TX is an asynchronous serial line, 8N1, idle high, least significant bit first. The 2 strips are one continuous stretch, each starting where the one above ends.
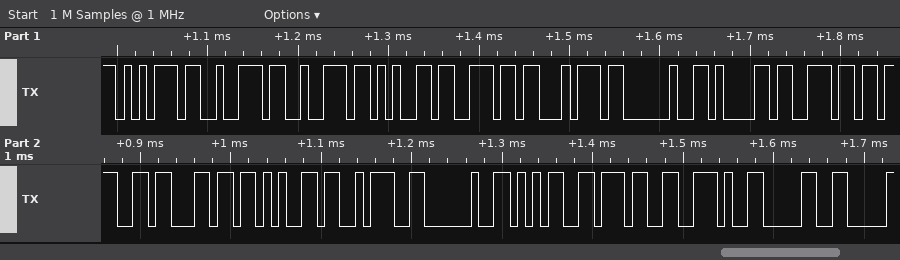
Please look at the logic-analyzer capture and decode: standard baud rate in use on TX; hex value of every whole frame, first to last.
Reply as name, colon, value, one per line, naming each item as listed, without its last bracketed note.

standard baud rate in use on TX: 115200 baud
hex value of every whole frame, first to last: 75 72 72 65 6E 74 20 61 6E 67 6C 65 3A 20 35 37 2E 30
